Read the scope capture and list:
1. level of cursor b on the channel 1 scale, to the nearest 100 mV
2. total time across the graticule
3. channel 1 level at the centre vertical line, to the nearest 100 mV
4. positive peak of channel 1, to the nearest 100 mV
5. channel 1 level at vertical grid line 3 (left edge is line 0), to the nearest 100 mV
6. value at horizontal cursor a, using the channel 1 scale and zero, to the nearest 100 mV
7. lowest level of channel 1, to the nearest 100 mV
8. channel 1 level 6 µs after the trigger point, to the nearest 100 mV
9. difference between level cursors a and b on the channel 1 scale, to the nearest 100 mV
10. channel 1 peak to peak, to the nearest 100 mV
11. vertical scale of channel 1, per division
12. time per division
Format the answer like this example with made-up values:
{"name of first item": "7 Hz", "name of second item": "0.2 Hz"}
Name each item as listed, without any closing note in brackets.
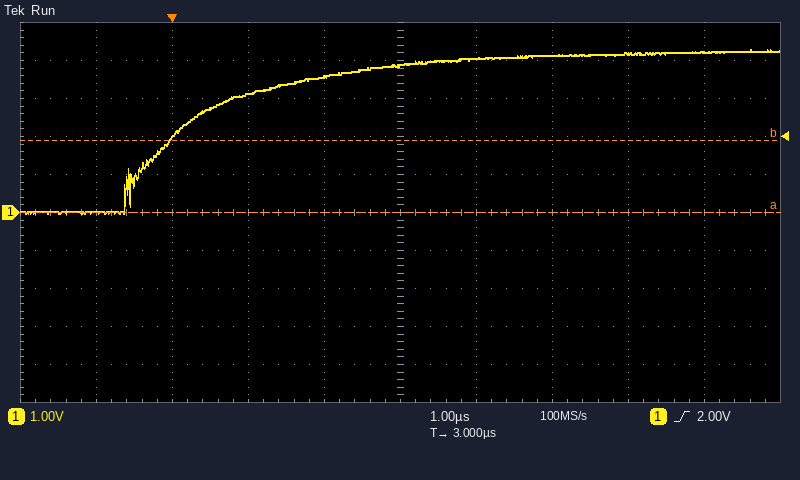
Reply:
{"level of cursor b on the channel 1 scale, to the nearest 100 mV": "1.9 V", "total time across the graticule": "10 µs", "channel 1 level at the centre vertical line, to the nearest 100 mV": "3.9 V", "positive peak of channel 1, to the nearest 100 mV": "4.3 V", "channel 1 level at vertical grid line 3 (left edge is line 0), to the nearest 100 mV": "3.1 V", "value at horizontal cursor a, using the channel 1 scale and zero, to the nearest 100 mV": "0.0 V", "lowest level of channel 1, to the nearest 100 mV": "0.0 V", "channel 1 level 6 µs after the trigger point, to the nearest 100 mV": "4.2 V", "difference between level cursors a and b on the channel 1 scale, to the nearest 100 mV": "1.9 V", "channel 1 peak to peak, to the nearest 100 mV": "4.3 V", "vertical scale of channel 1, per division": "1 V", "time per division": "1 µs"}
